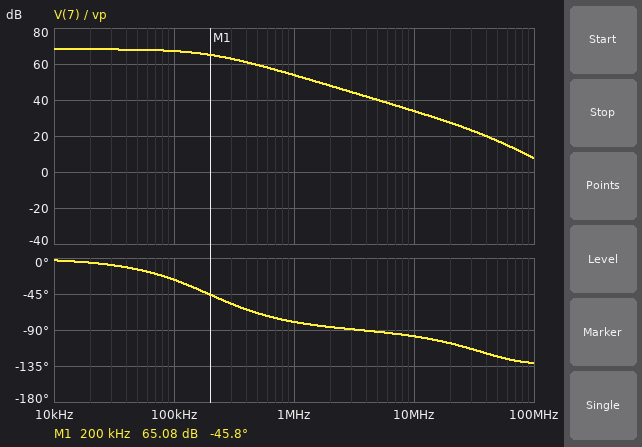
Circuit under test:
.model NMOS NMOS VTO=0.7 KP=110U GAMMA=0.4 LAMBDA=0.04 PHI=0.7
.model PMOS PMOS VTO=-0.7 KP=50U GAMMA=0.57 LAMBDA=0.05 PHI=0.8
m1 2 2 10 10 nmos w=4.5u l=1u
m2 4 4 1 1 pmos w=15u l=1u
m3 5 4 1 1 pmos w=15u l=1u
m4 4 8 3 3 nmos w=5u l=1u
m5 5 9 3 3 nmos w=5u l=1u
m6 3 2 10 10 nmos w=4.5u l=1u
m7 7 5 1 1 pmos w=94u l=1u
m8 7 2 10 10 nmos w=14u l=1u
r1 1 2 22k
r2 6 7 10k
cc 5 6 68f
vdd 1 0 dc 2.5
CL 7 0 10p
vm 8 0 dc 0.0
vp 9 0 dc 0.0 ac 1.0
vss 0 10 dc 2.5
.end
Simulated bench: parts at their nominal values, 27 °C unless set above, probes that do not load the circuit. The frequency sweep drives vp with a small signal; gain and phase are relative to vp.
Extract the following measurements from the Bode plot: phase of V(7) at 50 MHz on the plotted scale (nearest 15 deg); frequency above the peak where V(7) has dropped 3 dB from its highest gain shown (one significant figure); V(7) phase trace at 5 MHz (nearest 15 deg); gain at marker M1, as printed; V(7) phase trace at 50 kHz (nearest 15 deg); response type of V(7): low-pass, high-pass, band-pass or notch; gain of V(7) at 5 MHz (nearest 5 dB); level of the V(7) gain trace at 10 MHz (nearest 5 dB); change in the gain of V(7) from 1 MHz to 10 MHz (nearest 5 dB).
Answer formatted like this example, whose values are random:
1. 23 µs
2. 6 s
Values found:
1. -120 deg
2. 200 kHz
3. -90 deg
4. 65.08 dB
5. -15 deg
6. low-pass
7. 40 dB
8. 35 dB
9. -20 dB
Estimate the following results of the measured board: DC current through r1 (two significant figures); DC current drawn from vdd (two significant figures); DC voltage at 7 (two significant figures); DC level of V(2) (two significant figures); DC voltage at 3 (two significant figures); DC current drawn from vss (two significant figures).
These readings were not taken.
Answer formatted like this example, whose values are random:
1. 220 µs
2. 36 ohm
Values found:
1. 160 µA
2. 840 µA
3. 300 mV
4. -1.0 V
5. -1.2 V
6. 840 µA
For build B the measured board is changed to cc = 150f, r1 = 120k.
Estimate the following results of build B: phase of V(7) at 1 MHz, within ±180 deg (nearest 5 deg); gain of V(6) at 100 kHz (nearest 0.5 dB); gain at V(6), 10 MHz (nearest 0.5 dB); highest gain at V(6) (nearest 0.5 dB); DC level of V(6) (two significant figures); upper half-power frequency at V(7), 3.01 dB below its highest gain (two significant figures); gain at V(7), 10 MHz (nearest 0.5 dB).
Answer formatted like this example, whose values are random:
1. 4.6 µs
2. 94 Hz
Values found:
1. -90 deg
2. 62.5 dB
3. 22.0 dB
4. 81.5 dB
5. 570 mV
6. 11 kHz
7. 21.5 dB
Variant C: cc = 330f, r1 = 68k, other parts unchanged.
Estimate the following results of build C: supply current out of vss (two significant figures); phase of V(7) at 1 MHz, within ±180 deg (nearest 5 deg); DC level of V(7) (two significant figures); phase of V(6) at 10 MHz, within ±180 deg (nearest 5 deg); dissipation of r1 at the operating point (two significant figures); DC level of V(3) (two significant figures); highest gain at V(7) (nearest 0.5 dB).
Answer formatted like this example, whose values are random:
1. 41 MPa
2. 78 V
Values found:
1. 300 µA
2. -90 deg
3. 500 mV
4. -115 deg
5. 220 µW
6. -1.0 V
7. 77.0 dB
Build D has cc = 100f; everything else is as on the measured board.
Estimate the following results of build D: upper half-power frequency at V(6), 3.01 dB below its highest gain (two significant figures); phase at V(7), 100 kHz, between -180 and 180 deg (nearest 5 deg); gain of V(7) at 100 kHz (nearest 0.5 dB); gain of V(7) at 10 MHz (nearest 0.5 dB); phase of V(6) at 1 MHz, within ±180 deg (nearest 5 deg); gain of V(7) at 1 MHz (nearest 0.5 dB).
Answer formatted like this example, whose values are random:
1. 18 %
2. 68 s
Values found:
1. 150 kHz
2. -35 deg
3. 66.5 dB
4. 31.5 dB
5. -85 deg
6. 51.5 dB
